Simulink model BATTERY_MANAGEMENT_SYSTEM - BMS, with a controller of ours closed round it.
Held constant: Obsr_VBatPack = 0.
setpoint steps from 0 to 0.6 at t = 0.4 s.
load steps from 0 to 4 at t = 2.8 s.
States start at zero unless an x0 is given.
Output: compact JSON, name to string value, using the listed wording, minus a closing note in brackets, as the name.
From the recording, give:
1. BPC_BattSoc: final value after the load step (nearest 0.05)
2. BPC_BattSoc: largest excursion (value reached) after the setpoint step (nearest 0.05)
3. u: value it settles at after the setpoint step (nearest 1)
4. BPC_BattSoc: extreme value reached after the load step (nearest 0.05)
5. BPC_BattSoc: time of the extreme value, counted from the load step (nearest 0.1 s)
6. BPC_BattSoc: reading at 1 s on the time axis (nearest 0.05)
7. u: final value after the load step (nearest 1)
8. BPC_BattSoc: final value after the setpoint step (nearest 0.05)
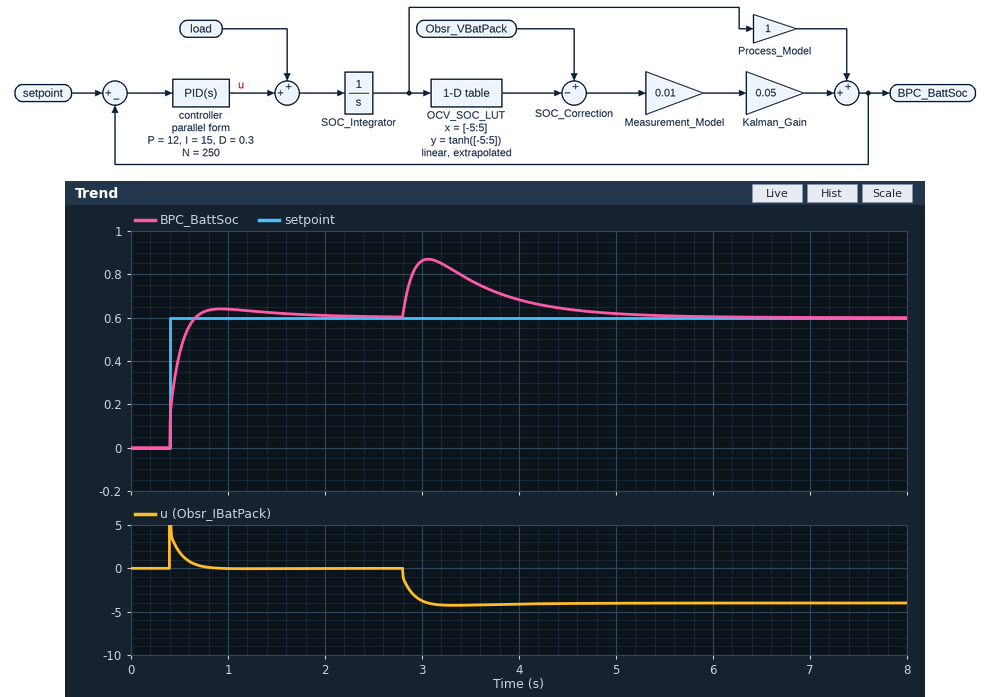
{"BPC_BattSoc: final value after the load step": "0.60", "BPC_BattSoc: largest excursion (value reached) after the setpoint step": "0.65", "u: value it settles at after the setpoint step": "0", "BPC_BattSoc: extreme value reached after the load step": "0.85", "BPC_BattSoc: time of the extreme value, counted from the load step": "0.3 s", "BPC_BattSoc: reading at 1 s on the time axis": "0.65", "u: final value after the load step": "-4", "BPC_BattSoc: final value after the setpoint step": "0.60"}
